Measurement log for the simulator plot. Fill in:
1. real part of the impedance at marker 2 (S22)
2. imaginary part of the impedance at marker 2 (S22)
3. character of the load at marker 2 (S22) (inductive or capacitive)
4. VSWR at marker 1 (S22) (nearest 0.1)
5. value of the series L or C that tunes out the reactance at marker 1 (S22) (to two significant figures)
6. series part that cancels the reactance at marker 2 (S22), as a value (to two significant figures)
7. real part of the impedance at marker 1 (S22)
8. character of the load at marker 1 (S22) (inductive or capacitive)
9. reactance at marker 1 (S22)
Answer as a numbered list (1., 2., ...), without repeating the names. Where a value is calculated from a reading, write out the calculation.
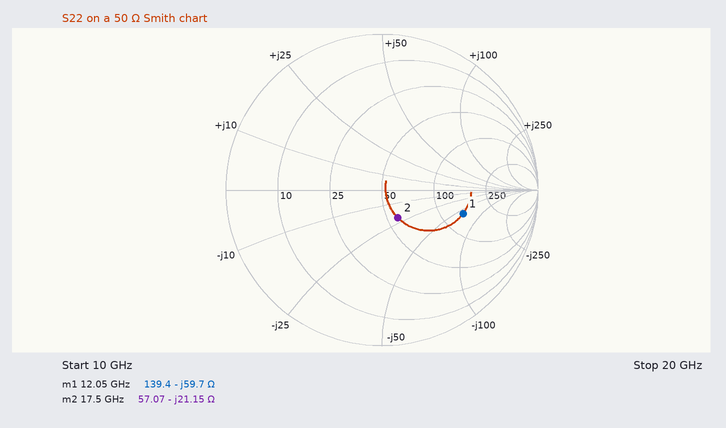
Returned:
1. 57.07 Ω
2. -21.15 Ω
3. capacitive
4. 3.4
5. L = 59.7 Ω/(2π × 12.05 GHz) ≈ 789 pH, so 790 pH to two significant figures
6. L = 21.15 Ω/(2π × 17.5 GHz) ≈ 192 pH, so 190 pH to two significant figures
7. 139.4 Ω
8. capacitive
9. -59.7 Ω
